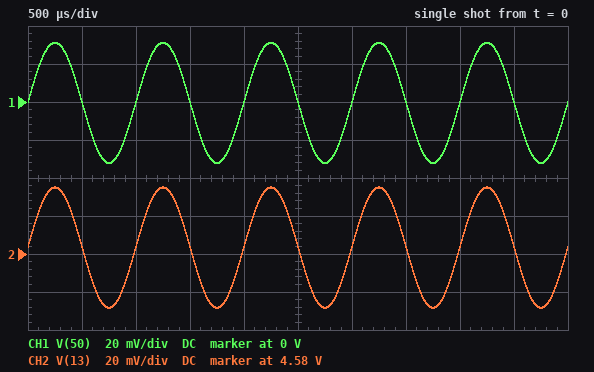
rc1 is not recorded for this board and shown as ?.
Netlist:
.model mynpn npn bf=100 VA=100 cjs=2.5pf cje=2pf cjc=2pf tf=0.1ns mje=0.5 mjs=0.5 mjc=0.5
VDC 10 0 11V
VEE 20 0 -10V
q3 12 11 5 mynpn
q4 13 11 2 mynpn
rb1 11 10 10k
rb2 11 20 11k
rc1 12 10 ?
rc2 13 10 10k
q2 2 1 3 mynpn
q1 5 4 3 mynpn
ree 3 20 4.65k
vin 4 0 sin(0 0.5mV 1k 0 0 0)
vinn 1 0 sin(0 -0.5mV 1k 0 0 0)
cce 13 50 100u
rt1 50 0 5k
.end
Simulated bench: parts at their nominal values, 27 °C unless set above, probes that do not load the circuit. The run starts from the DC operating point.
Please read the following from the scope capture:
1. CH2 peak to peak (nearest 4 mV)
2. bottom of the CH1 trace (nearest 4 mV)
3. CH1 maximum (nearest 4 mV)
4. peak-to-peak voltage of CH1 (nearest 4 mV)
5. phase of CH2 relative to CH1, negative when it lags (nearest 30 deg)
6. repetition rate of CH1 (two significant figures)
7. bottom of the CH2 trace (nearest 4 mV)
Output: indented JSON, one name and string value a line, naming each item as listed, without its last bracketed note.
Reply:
{
  "CH2 peak to peak": "64 mV",
  "bottom of the CH1 trace": "-32 mV",
  "CH1 maximum": "32 mV",
  "peak-to-peak voltage of CH1": "64 mV",
  "phase of CH2 relative to CH1, negative when it lags": "0 deg",
  "repetition rate of CH1": "1.0 kHz",
  "bottom of the CH2 trace": "4.552 V"
}
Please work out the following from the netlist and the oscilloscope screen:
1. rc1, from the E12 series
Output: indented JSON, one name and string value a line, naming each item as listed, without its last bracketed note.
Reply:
{
  "rc1, from the E12 series": "33 kΩ"
}
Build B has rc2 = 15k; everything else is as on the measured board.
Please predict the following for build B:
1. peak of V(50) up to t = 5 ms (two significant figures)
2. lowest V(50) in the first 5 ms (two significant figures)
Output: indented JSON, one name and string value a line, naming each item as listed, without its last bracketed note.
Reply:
{
  "peak of V(50) up to t = 5 ms": "34 mV",
  "lowest V(50) in the first 5 ms": "-35 mV"
}
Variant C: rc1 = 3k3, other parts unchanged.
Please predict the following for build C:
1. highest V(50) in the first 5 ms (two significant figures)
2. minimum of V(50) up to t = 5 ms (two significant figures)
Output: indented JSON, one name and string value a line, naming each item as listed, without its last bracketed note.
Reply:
{
  "highest V(50) in the first 5 ms": "63 mV",
  "minimum of V(50) up to t = 5 ms": "-63 mV"
}
